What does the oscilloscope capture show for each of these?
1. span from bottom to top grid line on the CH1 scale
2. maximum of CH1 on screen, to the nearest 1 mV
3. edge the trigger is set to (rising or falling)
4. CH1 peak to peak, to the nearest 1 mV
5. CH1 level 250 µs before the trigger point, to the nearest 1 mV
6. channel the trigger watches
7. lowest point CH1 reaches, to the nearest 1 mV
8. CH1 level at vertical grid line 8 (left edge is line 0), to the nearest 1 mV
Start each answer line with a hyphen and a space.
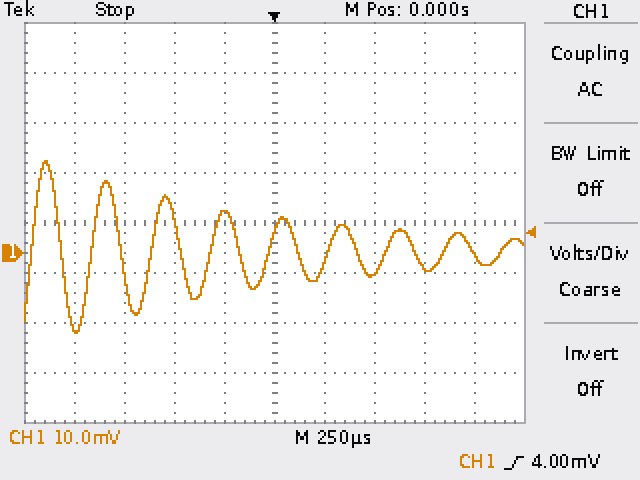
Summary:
- 80 mV
- 18 mV
- rising
- 34 mV
- 8 mV
- CH1
- -16 mV
- -3 mV
